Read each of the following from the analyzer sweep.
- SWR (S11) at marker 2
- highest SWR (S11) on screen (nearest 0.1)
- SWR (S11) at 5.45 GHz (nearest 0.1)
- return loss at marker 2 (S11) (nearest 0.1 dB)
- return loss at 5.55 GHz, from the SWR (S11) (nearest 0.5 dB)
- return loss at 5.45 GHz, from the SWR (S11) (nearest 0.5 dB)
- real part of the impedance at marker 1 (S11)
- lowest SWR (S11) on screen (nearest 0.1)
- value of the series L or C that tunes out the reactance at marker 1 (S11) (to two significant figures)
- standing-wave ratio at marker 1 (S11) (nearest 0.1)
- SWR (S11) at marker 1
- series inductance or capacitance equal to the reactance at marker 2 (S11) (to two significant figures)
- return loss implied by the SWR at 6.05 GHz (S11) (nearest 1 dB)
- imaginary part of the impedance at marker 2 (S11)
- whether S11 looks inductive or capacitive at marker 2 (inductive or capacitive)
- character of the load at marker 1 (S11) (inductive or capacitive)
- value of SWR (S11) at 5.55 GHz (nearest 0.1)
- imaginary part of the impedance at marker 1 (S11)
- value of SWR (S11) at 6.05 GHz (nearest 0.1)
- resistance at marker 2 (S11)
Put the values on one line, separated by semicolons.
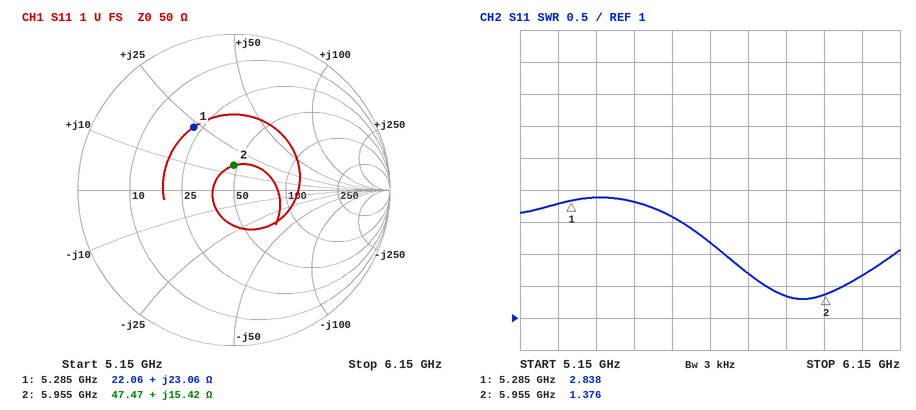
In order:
1.376; 2.9; 2.8; 16.0 dB; 7.0 dB; 6.5 dB; 22.06 Ω; 1.3; 1.3 pF; 2.8; 2.838; 410 pH; 12 dB; +15.42 Ω; inductive; inductive; 2.6; +23.06 Ω; 1.7; 47.47 Ω
